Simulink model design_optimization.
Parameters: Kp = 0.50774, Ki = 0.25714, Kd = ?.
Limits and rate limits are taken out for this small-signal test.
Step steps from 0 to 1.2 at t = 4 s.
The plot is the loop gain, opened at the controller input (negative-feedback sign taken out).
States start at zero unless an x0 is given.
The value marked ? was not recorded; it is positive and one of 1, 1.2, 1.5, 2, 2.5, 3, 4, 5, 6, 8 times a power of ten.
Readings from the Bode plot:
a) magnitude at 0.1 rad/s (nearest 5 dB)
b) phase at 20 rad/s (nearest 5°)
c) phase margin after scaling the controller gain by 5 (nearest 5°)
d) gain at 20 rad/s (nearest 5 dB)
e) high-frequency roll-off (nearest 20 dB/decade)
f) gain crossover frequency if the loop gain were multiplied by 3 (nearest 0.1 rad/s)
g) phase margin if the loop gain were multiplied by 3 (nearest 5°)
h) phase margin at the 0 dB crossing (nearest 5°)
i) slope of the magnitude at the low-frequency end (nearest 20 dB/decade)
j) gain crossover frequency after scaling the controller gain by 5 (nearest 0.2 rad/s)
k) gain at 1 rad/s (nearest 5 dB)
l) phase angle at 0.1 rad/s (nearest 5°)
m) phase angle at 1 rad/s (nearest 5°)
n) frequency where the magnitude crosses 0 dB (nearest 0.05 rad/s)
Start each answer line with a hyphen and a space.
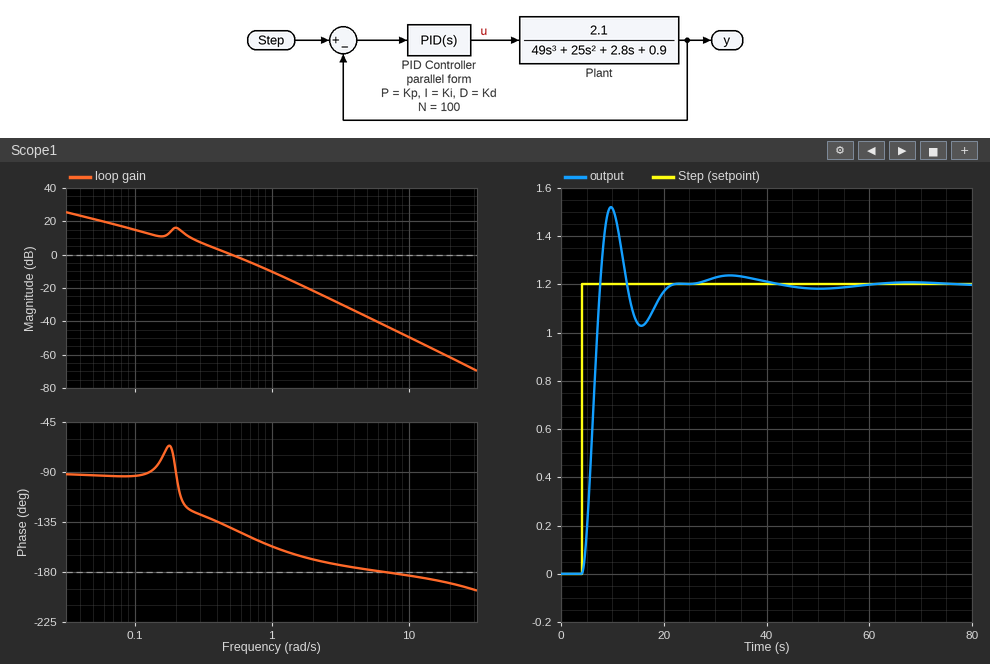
- 15 dB
- -190°
- 20°
- -60 dB
- -40 dB/decade
- 1.0 rad/s
- 25°
- 40°
- -20 dB/decade
- 1.2 rad/s
- -10 dB
- -95°
- -155°
- 0.50 rad/s
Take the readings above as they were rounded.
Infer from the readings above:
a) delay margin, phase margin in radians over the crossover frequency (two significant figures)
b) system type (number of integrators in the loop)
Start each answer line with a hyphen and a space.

- 1.4 s
- 1
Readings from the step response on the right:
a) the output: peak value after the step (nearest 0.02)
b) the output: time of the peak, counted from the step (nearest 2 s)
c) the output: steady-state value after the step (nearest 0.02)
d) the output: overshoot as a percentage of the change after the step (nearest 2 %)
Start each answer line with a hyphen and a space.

- 1.52
- 6 s
- 1.20
- 26 %
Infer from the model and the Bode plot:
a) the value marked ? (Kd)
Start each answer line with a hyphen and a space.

- 8
